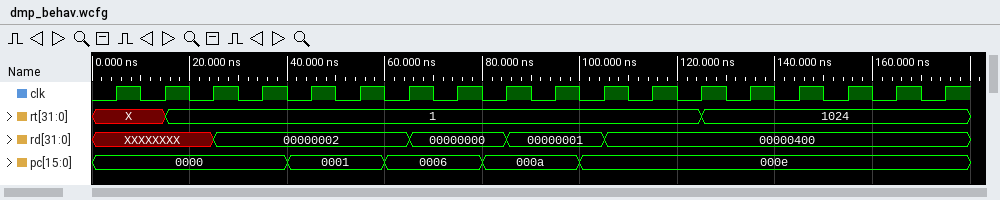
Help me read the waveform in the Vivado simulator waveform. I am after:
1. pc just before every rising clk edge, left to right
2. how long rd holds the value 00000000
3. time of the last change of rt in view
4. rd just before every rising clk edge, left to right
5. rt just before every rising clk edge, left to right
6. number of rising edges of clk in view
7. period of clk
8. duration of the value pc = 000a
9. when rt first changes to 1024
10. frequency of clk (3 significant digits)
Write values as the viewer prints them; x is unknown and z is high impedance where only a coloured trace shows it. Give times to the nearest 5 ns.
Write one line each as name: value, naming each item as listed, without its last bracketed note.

pc just before every rising clk edge, left to right: 0000, 0000, 0000, 0000, 0001, 0001, 0006, 0006, 000a, 000a, 000e, 000e, 000e, 000e, 000e, 000e, 000e, 000e
how long rd holds the value 00000000: 20 ns
time of the last change of rt in view: 125 ns
rd just before every rising clk edge, left to right: XXXXXXXX, XXXXXXXX, XXXXXXXX, 00000002, 00000002, 00000002, 00000002, 00000000, 00000000, 00000001, 00000001, 00000400, 00000400, 00000400, 00000400, 00000400, 00000400, 00000400
rt just before every rising clk edge, left to right: X, X, 1, 1, 1, 1, 1, 1, 1, 1, 1, 1, 1, 1024, 1024, 1024, 1024, 1024
number of rising edges of clk in view: 18
period of clk: 10 ns
duration of the value pc = 000a: 20 ns
when rt first changes to 1024: 125 ns
frequency of clk: 100 MHz
